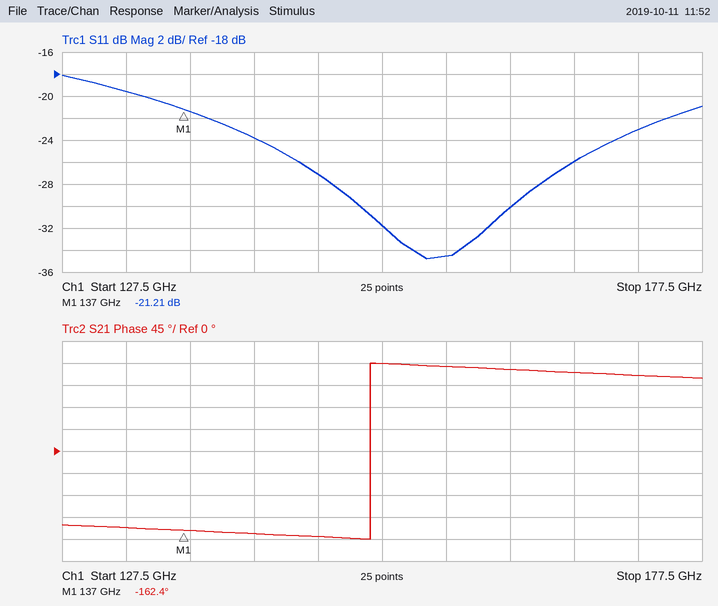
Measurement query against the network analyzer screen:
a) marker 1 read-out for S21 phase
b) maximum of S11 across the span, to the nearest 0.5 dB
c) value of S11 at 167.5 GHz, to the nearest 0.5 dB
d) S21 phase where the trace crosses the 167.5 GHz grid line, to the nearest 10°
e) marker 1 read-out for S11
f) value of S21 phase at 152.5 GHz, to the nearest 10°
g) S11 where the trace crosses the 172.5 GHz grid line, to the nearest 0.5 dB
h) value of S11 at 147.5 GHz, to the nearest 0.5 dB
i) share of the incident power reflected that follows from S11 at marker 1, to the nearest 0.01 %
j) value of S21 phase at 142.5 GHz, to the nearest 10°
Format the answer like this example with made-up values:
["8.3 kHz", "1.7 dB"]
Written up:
["-162.4°", "-18.0 dB", "-26.0 dB", "160°", "-21.21 dB", "180°", "-23.0 dB", "-27.0 dB", "0.76 %", "-170°"]
